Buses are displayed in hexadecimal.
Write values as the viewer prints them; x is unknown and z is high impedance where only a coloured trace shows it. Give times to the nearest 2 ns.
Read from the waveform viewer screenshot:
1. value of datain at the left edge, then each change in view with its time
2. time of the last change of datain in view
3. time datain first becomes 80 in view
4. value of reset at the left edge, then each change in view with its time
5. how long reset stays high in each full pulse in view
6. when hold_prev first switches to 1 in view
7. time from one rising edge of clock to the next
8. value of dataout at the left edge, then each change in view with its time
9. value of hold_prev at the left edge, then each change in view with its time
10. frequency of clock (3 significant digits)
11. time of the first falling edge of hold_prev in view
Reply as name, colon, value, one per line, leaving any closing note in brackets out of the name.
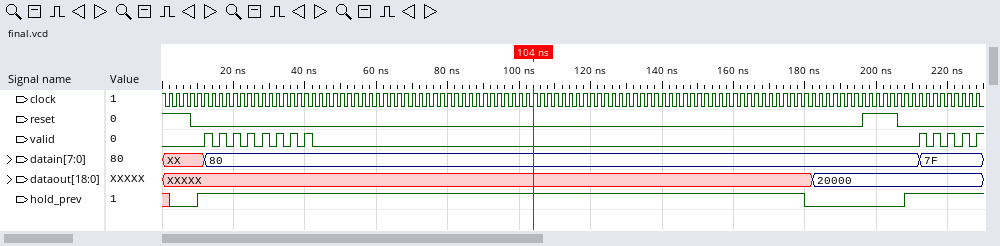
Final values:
value of datain at the left edge, then each change in view with its time: XX, 80 at 12 ns, 7F at 212 ns
time of the last change of datain in view: 212 ns
time datain first becomes 80 in view: 12 ns
value of reset at the left edge, then each change in view with its time: 1, 0 at 8 ns, 1 at 196 ns, 0 at 206 ns
how long reset stays high in each full pulse in view: 10 ns
when hold_prev first switches to 1 in view: 10 ns
time from one rising edge of clock to the next: 2 ns
value of dataout at the left edge, then each change in view with its time: XXXXX, 20000 at 182 ns
value of hold_prev at the left edge, then each change in view with its time: x, 0 at 2 ns, 1 at 10 ns, 0 at 180 ns, 1 at 208 ns
frequency of clock: 500 MHz
time of the first falling edge of hold_prev in view: 180 ns
